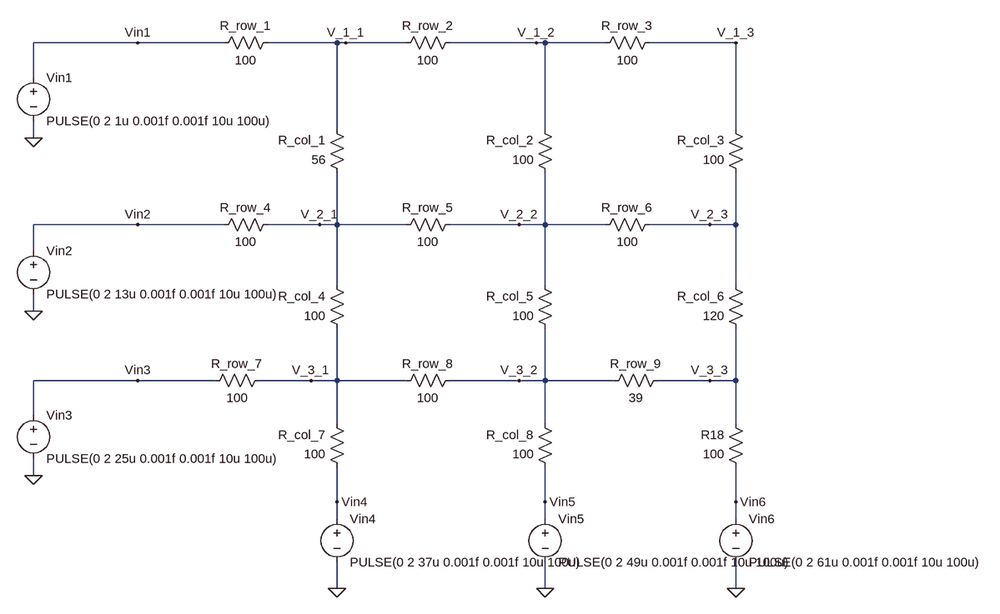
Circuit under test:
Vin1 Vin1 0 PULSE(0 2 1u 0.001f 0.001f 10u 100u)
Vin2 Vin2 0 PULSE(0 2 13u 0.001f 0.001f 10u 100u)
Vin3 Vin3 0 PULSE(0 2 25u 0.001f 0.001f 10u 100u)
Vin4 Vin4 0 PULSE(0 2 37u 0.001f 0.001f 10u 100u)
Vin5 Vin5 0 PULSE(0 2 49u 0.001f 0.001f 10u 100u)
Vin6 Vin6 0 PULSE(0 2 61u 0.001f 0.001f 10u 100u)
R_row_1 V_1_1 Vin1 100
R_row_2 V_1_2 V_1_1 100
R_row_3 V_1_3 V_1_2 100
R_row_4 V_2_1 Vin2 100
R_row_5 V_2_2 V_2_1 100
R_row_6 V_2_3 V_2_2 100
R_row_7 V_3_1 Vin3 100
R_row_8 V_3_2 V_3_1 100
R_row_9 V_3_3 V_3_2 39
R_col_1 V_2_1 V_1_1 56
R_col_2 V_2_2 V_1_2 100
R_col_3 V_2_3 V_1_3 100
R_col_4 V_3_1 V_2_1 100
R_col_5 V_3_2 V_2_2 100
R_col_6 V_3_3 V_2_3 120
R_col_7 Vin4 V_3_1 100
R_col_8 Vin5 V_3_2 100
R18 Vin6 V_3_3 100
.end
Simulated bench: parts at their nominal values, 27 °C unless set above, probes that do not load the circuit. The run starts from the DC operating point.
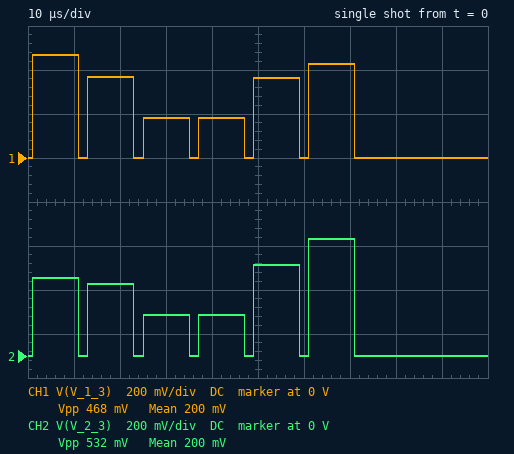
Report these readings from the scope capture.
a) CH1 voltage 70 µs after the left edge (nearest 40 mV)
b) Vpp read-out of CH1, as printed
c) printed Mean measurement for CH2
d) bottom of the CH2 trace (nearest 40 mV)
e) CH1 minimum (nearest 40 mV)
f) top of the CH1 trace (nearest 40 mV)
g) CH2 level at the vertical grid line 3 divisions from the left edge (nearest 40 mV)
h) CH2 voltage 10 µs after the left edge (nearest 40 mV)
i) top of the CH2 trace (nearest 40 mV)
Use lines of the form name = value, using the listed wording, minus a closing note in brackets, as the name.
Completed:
CH1 voltage 70 µs after the left edge = 440 mV
Vpp read-out of CH1, as printed = 468 mV
printed Mean measurement for CH2 = 200 mV
bottom of the CH2 trace = 0 V
CH1 minimum = 0 V
top of the CH1 trace = 480 mV
CH2 level at the vertical grid line 3 divisions from the left edge = 200 mV
CH2 voltage 10 µs after the left edge = 360 mV
top of the CH2 trace = 520 mV
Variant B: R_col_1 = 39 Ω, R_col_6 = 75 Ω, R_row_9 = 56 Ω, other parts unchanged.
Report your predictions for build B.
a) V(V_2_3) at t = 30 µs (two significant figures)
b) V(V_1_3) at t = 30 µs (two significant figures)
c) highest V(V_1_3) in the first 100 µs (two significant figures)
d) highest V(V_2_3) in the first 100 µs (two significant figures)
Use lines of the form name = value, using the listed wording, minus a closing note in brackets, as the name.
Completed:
V(V_2_3) at t = 30 µs = 180 mV
V(V_1_3) at t = 30 µs = 180 mV
highest V(V_1_3) in the first 100 µs = 490 mV
highest V(V_2_3) in the first 100 µs = 620 mV
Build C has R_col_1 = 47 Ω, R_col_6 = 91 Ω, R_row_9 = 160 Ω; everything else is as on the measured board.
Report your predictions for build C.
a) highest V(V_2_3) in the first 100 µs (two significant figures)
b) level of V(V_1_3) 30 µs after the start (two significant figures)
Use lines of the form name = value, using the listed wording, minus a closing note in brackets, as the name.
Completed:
highest V(V_2_3) in the first 100 µs = 670 mV
level of V(V_1_3) 30 µs after the start = 170 mV
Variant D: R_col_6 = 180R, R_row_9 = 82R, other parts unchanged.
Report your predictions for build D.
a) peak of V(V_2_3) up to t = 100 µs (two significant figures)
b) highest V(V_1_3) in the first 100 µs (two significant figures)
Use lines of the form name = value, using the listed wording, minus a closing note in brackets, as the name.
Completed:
peak of V(V_2_3) up to t = 100 µs = 510 mV
highest V(V_1_3) in the first 100 µs = 490 mV
